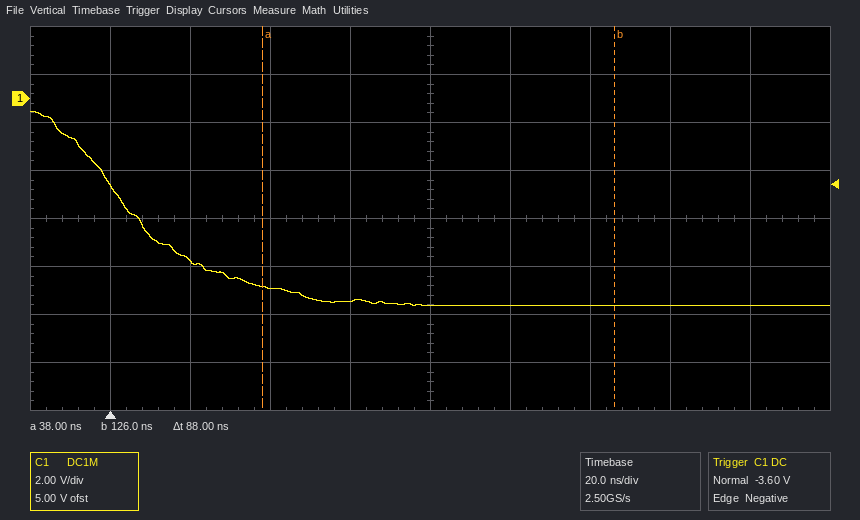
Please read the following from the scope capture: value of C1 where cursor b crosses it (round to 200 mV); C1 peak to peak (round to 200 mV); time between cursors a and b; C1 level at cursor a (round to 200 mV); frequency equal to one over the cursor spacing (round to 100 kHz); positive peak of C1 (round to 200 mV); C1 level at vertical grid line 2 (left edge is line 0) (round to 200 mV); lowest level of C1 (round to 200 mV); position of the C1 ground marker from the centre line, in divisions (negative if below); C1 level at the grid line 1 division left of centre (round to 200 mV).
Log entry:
-8.6 V
8.0 V
88 ns
-7.8 V
11.4 MHz
-600 mV
-6.8 V
-8.6 V
+2.5 div
-8.4 V
